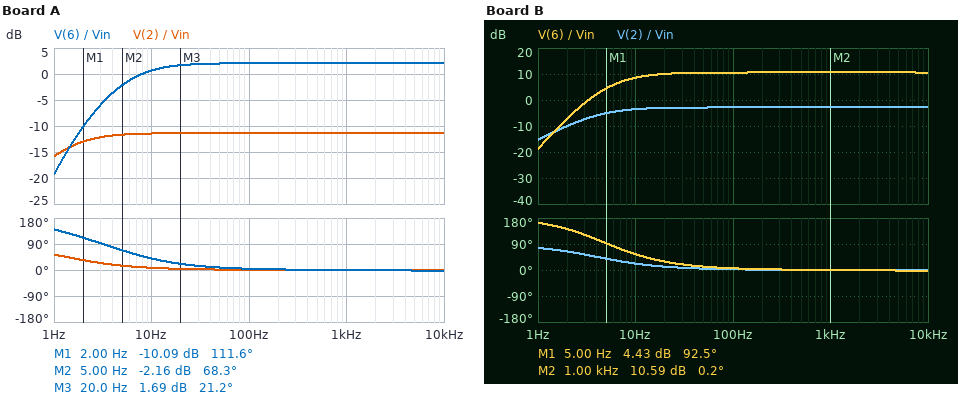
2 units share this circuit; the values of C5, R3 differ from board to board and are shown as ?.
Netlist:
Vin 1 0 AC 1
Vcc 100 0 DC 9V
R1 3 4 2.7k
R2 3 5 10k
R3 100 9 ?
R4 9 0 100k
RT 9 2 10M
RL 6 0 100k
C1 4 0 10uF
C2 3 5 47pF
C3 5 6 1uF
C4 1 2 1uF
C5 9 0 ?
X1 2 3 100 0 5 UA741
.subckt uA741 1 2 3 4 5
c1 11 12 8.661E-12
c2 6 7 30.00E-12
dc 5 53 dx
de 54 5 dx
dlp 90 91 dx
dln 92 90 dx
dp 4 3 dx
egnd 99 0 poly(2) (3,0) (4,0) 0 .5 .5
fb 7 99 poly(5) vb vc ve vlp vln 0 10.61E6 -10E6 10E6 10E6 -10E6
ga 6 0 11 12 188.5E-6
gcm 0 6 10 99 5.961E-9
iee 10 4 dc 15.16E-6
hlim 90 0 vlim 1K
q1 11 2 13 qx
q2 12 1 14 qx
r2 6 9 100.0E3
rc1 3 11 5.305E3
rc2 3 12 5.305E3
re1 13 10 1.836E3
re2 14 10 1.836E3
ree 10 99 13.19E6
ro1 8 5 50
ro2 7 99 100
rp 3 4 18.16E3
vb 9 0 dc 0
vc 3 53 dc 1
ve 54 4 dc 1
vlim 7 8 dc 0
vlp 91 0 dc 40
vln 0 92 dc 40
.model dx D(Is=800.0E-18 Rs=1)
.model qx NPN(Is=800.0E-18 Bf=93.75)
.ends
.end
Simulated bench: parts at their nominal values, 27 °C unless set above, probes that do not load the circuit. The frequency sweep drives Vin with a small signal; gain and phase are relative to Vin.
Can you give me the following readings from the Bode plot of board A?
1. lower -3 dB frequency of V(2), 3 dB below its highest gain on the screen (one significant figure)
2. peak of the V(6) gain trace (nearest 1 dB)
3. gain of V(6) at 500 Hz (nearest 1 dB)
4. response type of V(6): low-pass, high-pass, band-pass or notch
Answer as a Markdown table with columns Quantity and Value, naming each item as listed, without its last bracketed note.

| Quantity | Value |
|---|---|
| lower -3 dB frequency of V(2), 3 dB below its highest gain on the screen | 1 Hz |
| peak of the V(6) gain trace | 2 dB |
| gain of V(6) at 500 Hz | 2 dB |
| response type of V(6): low-pass, high-pass, band-pass or notch | high-pass |
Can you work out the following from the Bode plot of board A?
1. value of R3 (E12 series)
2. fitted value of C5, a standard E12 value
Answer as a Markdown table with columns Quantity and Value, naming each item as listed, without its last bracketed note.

| Quantity | Value |
|---|---|
| value of R3 | 47 kΩ |
| fitted value of C5, a standard E12 value | 2.7 µF |
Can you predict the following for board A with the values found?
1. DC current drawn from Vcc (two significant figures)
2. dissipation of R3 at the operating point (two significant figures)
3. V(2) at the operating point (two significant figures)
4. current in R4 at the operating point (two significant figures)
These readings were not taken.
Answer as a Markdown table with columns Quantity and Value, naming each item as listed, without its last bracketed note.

| Quantity | Value |
|---|---|
| DC current drawn from Vcc | 570 µA |
| dissipation of R3 at the operating point | 180 µW |
| V(2) at the operating point | 6.1 V |
| current in R4 at the operating point | 61 µA |
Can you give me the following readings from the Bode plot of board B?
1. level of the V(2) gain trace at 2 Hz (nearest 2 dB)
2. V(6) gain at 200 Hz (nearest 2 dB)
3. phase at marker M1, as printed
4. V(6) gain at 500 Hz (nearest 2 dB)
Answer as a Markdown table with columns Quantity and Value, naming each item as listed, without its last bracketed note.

| Quantity | Value |
|---|---|
| level of the V(2) gain trace at 2 Hz | -10 dB |
| V(6) gain at 200 Hz | 10 dB |
| phase at marker M1, as printed | 92.5 deg |
| V(6) gain at 500 Hz | 10 dB |
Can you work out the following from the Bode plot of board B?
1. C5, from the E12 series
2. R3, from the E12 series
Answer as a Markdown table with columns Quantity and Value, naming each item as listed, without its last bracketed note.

| Quantity | Value |
|---|---|
| C5, from the E12 series | 390 nF |
| R3, from the E12 series | 39 kΩ |
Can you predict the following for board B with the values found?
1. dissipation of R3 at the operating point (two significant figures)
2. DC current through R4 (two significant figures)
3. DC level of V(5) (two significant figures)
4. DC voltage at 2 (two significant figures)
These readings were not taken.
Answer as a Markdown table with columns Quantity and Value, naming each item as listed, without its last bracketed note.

| Quantity | Value |
|---|---|
| dissipation of R3 at the operating point | 160 µW |
| DC current through R4 | 65 µA |
| DC level of V(5) | 6.5 V |
| DC voltage at 2 | 6.5 V |
